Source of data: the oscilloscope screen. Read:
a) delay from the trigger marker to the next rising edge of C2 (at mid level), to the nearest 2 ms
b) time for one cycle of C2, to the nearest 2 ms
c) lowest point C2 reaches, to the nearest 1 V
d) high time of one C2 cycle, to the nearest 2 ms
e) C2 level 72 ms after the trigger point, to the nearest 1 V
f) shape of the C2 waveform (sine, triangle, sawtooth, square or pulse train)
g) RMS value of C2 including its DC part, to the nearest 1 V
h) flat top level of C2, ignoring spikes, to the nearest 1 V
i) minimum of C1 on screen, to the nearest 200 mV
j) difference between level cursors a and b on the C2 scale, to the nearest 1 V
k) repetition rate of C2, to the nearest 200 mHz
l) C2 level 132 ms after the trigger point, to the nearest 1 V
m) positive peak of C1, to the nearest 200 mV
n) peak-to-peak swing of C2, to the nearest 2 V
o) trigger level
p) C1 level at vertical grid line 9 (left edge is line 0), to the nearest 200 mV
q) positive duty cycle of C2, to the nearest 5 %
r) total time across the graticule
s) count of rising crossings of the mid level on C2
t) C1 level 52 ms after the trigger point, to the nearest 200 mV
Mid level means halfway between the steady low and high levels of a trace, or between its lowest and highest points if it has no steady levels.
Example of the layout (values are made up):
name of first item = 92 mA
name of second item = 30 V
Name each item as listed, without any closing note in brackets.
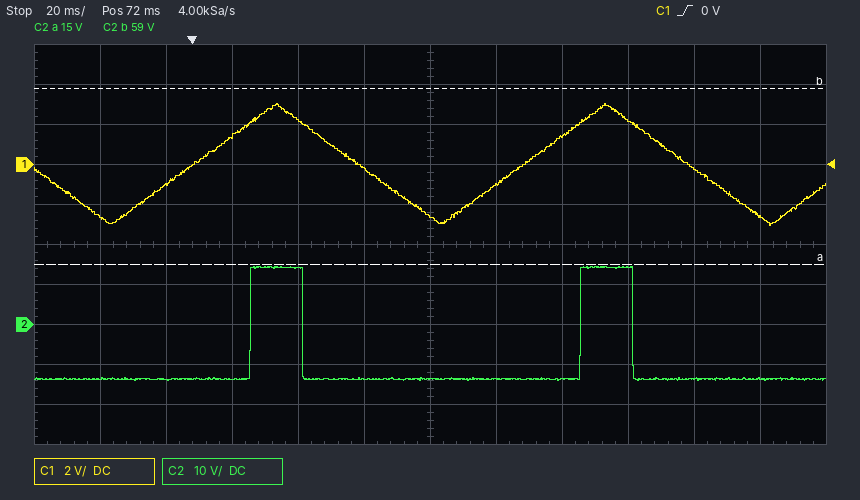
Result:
delay from the trigger marker to the next rising edge of C2 (at mid level), to the nearest 2 ms = 18 ms
time for one cycle of C2, to the nearest 2 ms = 100 ms
lowest point C2 reaches, to the nearest 1 V = -14 V
high time of one C2 cycle, to the nearest 2 ms = 16 ms
C2 level 72 ms after the trigger point, to the nearest 1 V = -14 V
shape of the C2 waveform = pulse train
RMS value of C2 including its DC part, to the nearest 1 V = 14 V
flat top level of C2, ignoring spikes, to the nearest 1 V = 14 V
minimum of C1 on screen, to the nearest 200 mV = -3.0 V
difference between level cursors a and b on the C2 scale, to the nearest 1 V = 44 V
repetition rate of C2, to the nearest 200 mHz = 10.0 Hz
C2 level 132 ms after the trigger point, to the nearest 1 V = 14 V
positive peak of C1, to the nearest 200 mV = 3.0 V
peak-to-peak swing of C2, to the nearest 2 V = 28 V
trigger level = 0 V
C1 level at vertical grid line 9 (left edge is line 0), to the nearest 200 mV = 2.2 V
positive duty cycle of C2, to the nearest 5 % = 15 %
total time across the graticule = 240 ms
count of rising crossings of the mid level on C2 = 2
C1 level 52 ms after the trigger point, to the nearest 200 mV = -200 mV
